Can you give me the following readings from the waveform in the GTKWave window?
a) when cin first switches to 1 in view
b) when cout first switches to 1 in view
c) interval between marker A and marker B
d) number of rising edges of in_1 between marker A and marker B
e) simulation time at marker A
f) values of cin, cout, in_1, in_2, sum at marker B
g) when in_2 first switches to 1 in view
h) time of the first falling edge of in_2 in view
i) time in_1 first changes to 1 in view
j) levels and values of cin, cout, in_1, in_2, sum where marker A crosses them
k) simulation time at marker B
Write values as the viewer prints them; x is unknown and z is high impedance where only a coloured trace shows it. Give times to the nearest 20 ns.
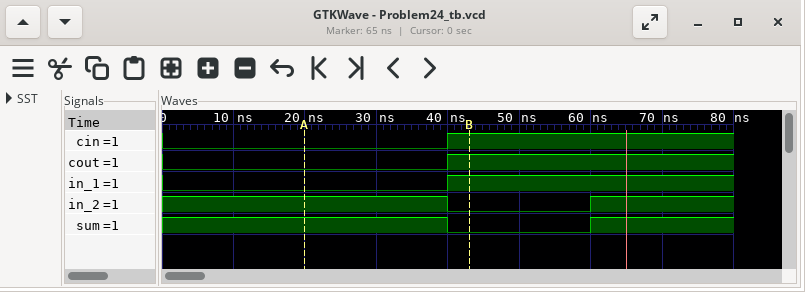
40 ns
40 ns
20 ns
1
20 ns
cin=1, cout=1, in_1=1, in_2=0, sum=0
60 ns
40 ns
40 ns
cin=0, cout=0, in_1=0, in_2=1, sum=1
40 ns
